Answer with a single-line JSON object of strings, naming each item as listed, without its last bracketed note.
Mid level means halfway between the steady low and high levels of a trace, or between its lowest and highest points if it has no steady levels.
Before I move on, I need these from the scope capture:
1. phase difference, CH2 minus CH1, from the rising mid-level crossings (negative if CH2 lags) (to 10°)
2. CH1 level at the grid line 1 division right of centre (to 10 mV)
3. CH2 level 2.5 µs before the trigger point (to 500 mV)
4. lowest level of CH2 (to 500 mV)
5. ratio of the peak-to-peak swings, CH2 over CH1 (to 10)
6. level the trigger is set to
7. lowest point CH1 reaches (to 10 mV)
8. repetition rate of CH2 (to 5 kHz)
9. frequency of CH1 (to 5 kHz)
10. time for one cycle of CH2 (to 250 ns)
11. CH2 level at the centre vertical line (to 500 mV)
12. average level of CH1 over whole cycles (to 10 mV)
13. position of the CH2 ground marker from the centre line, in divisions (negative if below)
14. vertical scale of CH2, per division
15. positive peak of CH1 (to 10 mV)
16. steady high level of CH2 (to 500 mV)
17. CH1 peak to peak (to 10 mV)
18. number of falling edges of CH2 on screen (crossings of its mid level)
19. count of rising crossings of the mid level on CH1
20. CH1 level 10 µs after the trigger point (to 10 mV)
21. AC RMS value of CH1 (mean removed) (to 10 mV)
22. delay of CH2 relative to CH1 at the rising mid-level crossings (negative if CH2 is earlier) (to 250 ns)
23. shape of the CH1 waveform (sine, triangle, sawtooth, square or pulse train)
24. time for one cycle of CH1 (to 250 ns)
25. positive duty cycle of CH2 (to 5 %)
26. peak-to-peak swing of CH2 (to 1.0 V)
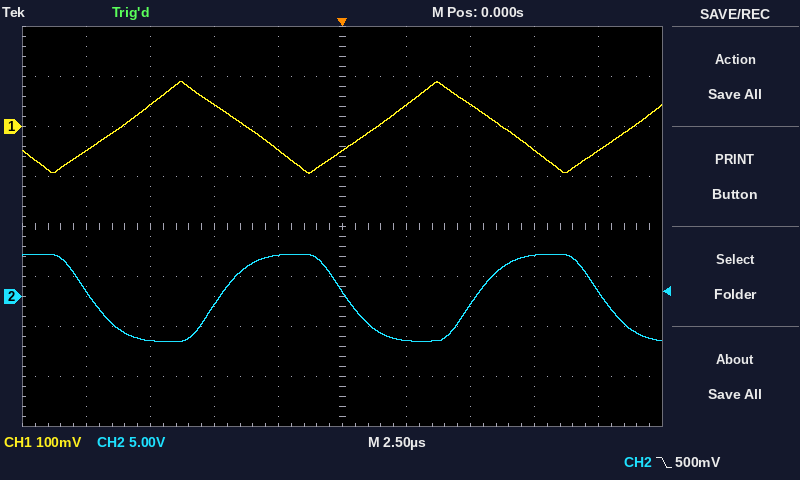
{"phase difference, CH2 minus CH1, from the rising mid-level crossings (negative if CH2 lags)": "-140°", "CH1 level at the grid line 1 division right of centre": "40 mV", "CH2 level 2.5 µs before the trigger point": "4.0 V", "lowest level of CH2": "-4.5 V", "ratio of the peak-to-peak swings, CH2 over CH1": "50", "level the trigger is set to": "500 mV", "lowest point CH1 reaches": "-90 mV", "repetition rate of CH2": "100 kHz", "frequency of CH1": "100 kHz", "time for one cycle of CH2": "10.00 µs", "CH2 level at the centre vertical line": "500 mV", "average level of CH1 over whole cycles": "0 mV", "position of the CH2 ground marker from the centre line, in divisions": "-1.4 div", "vertical scale of CH2, per division": "5 V", "positive peak of CH1": "90 mV", "steady high level of CH2": "4.0 V", "CH1 peak to peak": "180 mV", "number of falling edges of CH2 on screen": "3", "count of rising crossings of the mid level on CH1": "3", "CH1 level 10 µs after the trigger point": "-50 mV", "AC RMS value of CH1 (mean removed)": "50 mV", "delay of CH2 relative to CH1 at the rising mid-level crossings (negative if CH2 is earlier)": "+3.75 µs", "shape of the CH1 waveform": "triangle", "time for one cycle of CH1": "10.00 µs", "positive duty cycle of CH2": "50 %", "peak-to-peak swing of CH2": "9.0 V"}
